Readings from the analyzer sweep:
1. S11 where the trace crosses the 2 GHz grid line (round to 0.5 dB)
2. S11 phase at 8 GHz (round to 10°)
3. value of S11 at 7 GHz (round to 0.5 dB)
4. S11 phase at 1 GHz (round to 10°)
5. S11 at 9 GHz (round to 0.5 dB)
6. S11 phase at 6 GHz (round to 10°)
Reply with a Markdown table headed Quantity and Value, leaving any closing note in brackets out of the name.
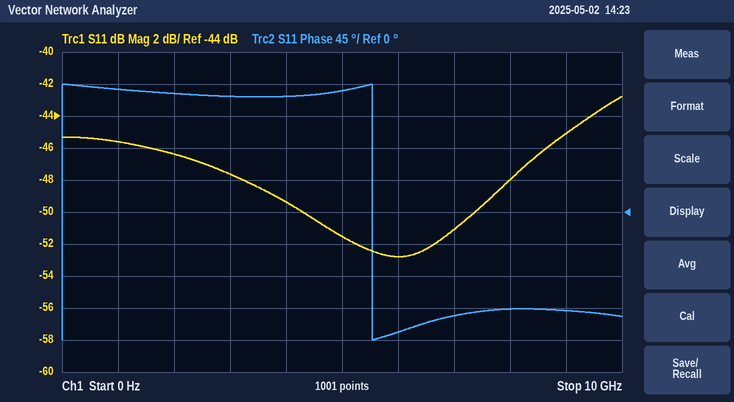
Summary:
| Quantity | Value |
|---|---|
| S11 where the trace crosses the 2 GHz grid line | -46.5 dB |
| S11 phase at 8 GHz | -140° |
| value of S11 at 7 GHz | -51.0 dB |
| S11 phase at 1 GHz | 170° |
| S11 at 9 GHz | -45.0 dB |
| S11 phase at 6 GHz | -170° |
